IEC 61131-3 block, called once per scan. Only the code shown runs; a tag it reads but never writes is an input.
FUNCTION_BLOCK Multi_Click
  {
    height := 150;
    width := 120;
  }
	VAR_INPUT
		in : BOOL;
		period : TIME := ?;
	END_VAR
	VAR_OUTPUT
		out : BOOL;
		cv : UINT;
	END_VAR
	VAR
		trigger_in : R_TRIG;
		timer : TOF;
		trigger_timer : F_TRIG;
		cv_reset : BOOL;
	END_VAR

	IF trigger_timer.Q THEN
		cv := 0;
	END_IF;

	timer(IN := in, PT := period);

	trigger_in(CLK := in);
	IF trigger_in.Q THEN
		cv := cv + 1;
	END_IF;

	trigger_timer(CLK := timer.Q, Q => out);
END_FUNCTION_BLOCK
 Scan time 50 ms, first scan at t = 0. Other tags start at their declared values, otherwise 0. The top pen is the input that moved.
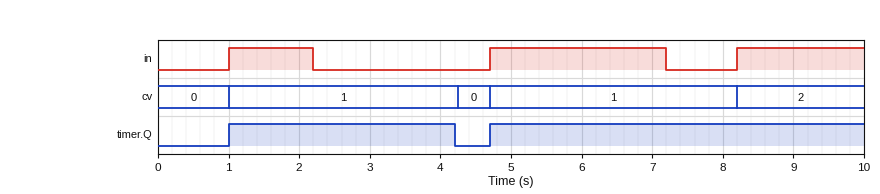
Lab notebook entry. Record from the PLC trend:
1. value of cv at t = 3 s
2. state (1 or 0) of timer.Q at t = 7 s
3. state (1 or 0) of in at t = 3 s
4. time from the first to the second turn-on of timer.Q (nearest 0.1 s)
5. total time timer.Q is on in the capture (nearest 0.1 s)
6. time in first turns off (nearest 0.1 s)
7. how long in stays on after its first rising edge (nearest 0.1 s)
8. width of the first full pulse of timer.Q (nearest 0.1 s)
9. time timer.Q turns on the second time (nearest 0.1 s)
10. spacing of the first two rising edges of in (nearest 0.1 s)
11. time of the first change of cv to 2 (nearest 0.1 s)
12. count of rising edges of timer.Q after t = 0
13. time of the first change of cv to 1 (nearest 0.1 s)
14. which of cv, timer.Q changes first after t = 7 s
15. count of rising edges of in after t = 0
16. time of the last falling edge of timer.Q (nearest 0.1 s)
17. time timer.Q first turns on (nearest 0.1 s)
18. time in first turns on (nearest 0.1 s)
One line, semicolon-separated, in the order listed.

1; 1; 0; 3.7 s; 8.5 s; 2.2 s; 1.2 s; 3.2 s; 4.7 s; 3.7 s; 8.2 s; 2; 1.0 s; cv; 3; 4.2 s; 1.0 s; 1.0 s
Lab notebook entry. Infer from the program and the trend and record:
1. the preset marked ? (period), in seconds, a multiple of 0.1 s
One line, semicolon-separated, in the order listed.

2.0 s
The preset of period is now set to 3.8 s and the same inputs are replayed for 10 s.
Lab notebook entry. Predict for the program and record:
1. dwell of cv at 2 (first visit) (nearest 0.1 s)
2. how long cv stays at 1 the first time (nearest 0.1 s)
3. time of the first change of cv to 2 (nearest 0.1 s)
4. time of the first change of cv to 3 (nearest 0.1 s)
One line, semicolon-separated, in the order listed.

3.5 s; 3.7 s; 4.7 s; 8.2 s
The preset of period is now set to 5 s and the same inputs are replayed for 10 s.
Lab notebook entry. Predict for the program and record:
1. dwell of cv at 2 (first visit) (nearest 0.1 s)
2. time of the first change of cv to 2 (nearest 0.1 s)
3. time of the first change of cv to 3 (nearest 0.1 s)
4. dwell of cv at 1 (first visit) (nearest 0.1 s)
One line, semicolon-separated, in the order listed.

3.5 s; 4.7 s; 8.2 s; 3.7 s
